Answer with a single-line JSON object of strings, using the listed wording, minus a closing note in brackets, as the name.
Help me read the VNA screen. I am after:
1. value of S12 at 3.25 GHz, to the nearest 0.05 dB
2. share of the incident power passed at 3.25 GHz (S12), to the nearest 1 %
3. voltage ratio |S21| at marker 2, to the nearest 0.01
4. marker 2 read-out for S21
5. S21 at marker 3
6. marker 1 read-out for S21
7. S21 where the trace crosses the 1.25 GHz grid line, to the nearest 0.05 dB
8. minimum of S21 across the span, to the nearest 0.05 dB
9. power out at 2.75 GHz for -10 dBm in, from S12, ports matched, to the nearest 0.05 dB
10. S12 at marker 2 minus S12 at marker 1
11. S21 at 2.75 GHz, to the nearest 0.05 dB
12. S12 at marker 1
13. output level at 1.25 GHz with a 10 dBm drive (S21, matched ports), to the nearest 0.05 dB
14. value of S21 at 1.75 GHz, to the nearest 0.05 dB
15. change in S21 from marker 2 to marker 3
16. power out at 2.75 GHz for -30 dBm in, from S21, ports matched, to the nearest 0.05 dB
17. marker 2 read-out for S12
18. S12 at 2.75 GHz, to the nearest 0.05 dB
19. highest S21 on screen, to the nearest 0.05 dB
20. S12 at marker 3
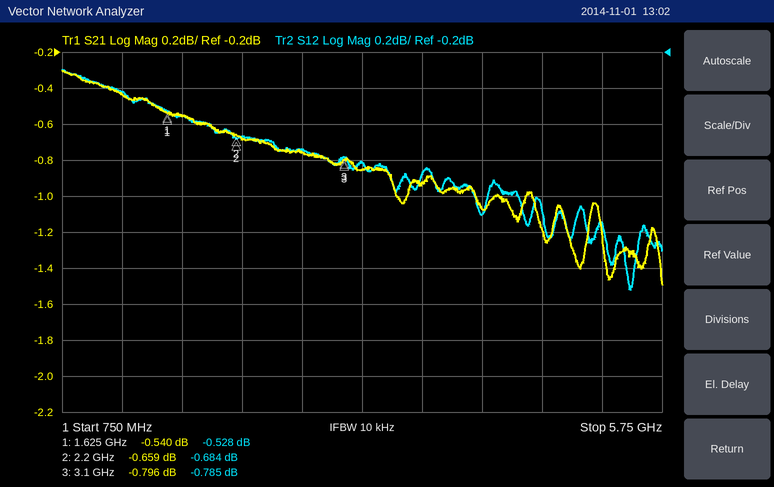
{"value of S12 at 3.25 GHz, to the nearest 0.05 dB": "-0.80 dB", "share of the incident power passed at 3.25 GHz (S12), to the nearest 1 %": "83 %", "voltage ratio |S21| at marker 2, to the nearest 0.01": "0.93", "marker 2 read-out for S21": "-0.659 dB", "S21 at marker 3": "-0.796 dB", "marker 1 read-out for S21": "-0.540 dB", "S21 where the trace crosses the 1.25 GHz grid line, to the nearest 0.05 dB": "-0.45 dB", "minimum of S21 across the span, to the nearest 0.05 dB": "-1.50 dB", "power out at 2.75 GHz for -10 dBm in, from S12, ports matched, to the nearest 0.05 dB": "-10.75 dBm", "S12 at marker 2 minus S12 at marker 1": "-0.156 dB", "S21 at 2.75 GHz, to the nearest 0.05 dB": "-0.75 dB", "S12 at marker 1": "-0.528 dB", "output level at 1.25 GHz with a 10 dBm drive (S21, matched ports), to the nearest 0.05 dB": "9.55 dBm", "value of S21 at 1.75 GHz, to the nearest 0.05 dB": "-0.55 dB", "change in S21 from marker 2 to marker 3": "-0.137 dB", "power out at 2.75 GHz for -30 dBm in, from S21, ports matched, to the nearest 0.05 dB": "-30.75 dBm", "marker 2 read-out for S12": "-0.684 dB", "S12 at 2.75 GHz, to the nearest 0.05 dB": "-0.75 dB", "highest S21 on screen, to the nearest 0.05 dB": "-0.30 dB", "S12 at marker 3": "-0.785 dB"}
